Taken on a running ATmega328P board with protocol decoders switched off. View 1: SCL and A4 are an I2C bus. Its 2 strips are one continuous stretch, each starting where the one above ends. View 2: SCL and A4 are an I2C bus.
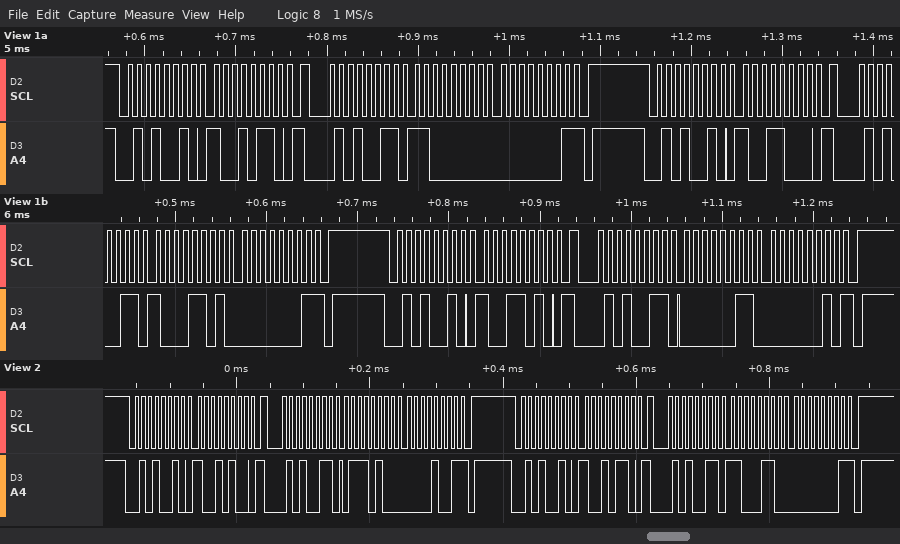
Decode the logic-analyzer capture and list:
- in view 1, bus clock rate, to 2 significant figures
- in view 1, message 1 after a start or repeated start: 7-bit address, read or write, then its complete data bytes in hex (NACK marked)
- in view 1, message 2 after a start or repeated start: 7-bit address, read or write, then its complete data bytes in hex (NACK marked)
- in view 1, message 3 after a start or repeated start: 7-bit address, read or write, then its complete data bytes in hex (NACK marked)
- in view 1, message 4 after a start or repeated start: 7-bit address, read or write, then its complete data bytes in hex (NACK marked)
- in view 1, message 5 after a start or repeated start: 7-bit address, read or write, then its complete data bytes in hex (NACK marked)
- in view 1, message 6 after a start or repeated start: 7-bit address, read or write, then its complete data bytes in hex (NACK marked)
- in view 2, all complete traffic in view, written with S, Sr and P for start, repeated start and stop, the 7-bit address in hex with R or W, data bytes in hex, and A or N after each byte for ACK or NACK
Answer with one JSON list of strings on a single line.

["100 kHz", "0x29 write: 96", "0x29 read: C0 01 NACK", "0x29 write: 98", "0x29 read: 8D 01 NACK", "0x29 write: 9A", "0x29 read: 03 02 NACK", "S 29W A 94 A Sr 29R A 74 A 09 N P S 29W A 96 A Sr 29R A C6 A 01 N P"]
